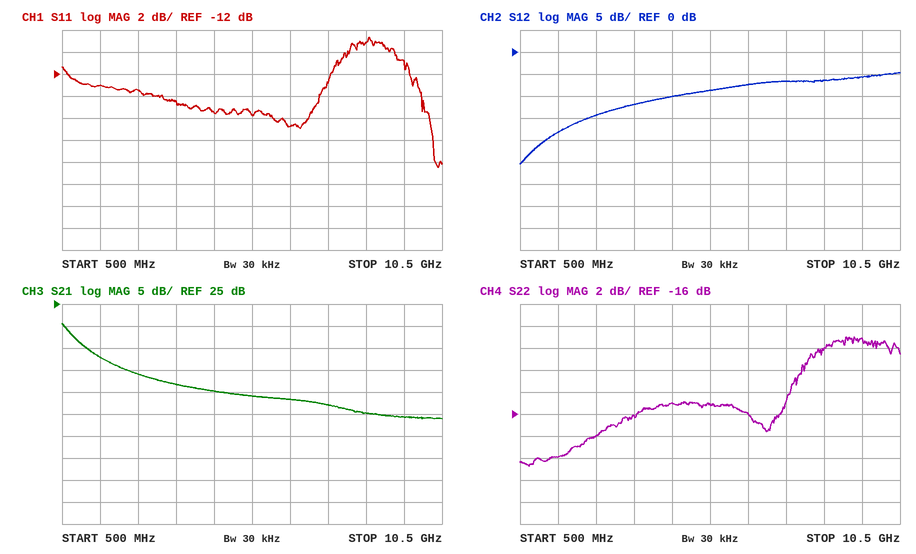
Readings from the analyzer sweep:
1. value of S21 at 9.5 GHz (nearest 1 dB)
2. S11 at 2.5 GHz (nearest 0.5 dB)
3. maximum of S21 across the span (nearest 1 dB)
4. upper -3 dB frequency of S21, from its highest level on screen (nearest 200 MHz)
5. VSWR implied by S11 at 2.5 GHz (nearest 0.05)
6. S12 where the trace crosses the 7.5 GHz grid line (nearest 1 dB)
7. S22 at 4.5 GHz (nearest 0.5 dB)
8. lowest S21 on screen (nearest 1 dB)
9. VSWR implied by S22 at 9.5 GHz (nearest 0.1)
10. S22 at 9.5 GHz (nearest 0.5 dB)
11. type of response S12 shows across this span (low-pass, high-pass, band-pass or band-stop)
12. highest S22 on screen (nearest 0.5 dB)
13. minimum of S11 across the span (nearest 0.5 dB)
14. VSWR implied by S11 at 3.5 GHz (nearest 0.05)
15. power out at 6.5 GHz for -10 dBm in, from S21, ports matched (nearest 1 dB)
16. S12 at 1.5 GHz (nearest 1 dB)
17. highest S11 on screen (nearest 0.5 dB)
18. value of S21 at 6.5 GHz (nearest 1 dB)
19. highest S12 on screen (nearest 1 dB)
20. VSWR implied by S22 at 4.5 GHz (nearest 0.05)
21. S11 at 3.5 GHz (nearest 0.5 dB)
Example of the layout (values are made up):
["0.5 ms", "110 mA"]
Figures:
["-1 dB", "-13.5 dB", "21 dB", "800 MHz", "1.55", "-7 dB", "-15.0 dB", "-1 dB", "2.1", "-9.0 dB", "high-pass", "-9.0 dB", "-20.5 dB", "1.45", "-7 dBm", "-18 dB", "-8.5 dB", "3 dB", "-5 dB", "1.45", "-14.5 dB"]
